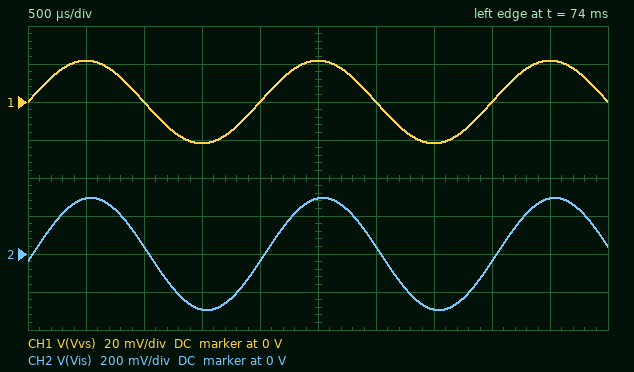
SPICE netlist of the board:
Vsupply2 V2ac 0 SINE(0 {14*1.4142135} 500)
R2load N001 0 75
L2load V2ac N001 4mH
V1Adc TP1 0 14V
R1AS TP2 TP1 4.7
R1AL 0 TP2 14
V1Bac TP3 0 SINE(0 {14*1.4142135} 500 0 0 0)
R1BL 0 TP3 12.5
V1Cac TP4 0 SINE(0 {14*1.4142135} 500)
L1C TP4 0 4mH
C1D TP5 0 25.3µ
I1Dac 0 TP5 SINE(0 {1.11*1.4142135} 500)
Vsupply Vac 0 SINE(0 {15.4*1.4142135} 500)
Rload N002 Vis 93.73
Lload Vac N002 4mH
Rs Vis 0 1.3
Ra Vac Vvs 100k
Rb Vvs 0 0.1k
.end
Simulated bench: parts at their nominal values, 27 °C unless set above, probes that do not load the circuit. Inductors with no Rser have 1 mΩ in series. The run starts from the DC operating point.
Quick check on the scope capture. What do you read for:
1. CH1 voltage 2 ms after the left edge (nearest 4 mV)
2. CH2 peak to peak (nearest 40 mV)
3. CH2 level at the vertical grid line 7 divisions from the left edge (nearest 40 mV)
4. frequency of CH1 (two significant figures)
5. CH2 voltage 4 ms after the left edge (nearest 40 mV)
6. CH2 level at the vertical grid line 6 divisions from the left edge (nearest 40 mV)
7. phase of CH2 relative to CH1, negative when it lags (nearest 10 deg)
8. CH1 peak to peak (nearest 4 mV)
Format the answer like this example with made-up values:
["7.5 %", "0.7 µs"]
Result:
["0 V", "600 mV", "-280 mV", "500 Hz", "-40 mV", "40 mV", "-10 deg", "44 mV"]
